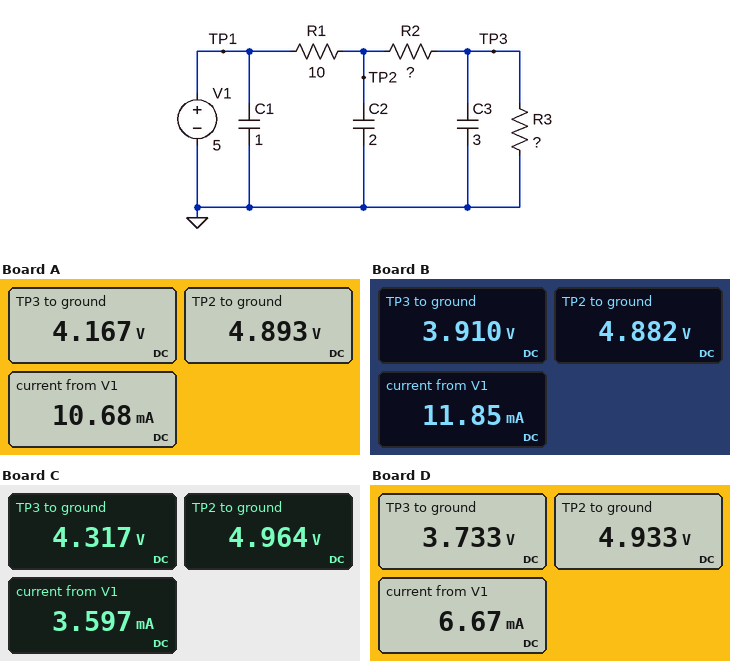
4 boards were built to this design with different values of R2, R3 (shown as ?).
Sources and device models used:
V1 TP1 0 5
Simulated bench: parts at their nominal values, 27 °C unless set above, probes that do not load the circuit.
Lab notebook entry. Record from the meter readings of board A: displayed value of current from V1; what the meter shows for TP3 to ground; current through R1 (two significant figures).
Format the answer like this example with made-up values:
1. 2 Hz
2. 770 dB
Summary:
1. 10.68 mA
2. 4.167 V
3. 11 mA
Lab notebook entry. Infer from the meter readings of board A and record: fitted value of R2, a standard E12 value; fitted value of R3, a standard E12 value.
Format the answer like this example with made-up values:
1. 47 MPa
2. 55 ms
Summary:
1. 68 Ω
2. 390 Ω
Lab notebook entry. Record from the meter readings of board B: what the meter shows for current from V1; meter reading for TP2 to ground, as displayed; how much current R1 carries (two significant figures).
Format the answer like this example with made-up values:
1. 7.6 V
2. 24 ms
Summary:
1. 11.85 mA
2. 4.882 V
3. 12 mA
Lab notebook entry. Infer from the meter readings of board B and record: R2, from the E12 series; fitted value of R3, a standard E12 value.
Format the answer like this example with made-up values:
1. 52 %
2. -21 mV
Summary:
1. 82 Ω
2. 330 Ω
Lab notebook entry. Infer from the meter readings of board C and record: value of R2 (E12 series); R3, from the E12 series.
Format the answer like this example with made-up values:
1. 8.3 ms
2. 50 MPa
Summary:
1. 180 Ω
2. 1.2 kΩ
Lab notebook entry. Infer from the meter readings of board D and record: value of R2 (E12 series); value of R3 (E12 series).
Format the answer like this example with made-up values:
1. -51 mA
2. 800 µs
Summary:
1. 180 Ω
2. 560 Ω
